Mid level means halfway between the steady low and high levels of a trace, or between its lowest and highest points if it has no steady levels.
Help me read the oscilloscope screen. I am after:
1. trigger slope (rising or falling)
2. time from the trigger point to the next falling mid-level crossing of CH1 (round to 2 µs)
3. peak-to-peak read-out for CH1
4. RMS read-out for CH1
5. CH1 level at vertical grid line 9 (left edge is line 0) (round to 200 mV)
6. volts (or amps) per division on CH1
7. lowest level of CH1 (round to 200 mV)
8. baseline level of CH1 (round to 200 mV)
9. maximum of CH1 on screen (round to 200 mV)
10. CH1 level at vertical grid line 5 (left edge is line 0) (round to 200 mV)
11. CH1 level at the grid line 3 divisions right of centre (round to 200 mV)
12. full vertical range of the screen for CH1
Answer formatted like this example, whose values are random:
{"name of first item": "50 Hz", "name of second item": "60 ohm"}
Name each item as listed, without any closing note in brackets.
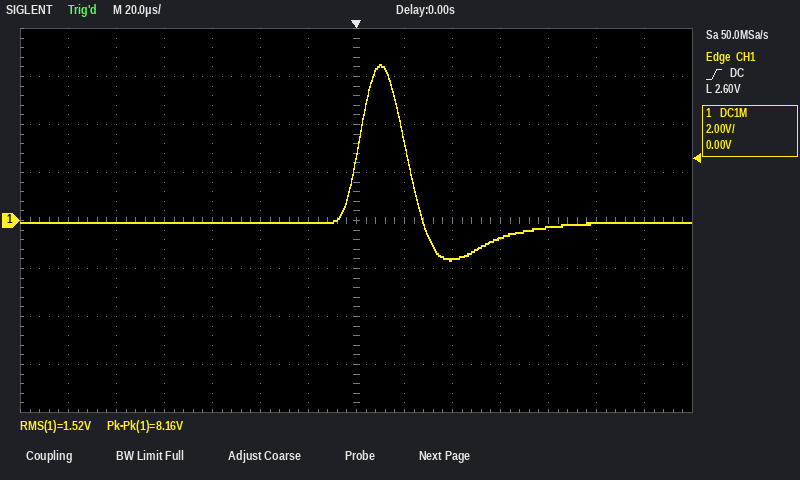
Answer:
{"trigger slope": "rising", "time from the trigger point to the next falling mid-level crossing of CH1": "22 µs", "peak-to-peak read-out for CH1": "8.16 V", "RMS read-out for CH1": "1.52 V", "CH1 level at vertical grid line 9 (left edge is line 0)": "-1.6 V", "volts (or amps) per division on CH1": "2 V", "lowest level of CH1": "-1.6 V", "baseline level of CH1": "0.0 V", "maximum of CH1 on screen": "6.4 V", "CH1 level at vertical grid line 5 (left edge is line 0)": "0.0 V", "CH1 level at the grid line 3 divisions right of centre": "-800 mV", "full vertical range of the screen for CH1": "16 V"}
